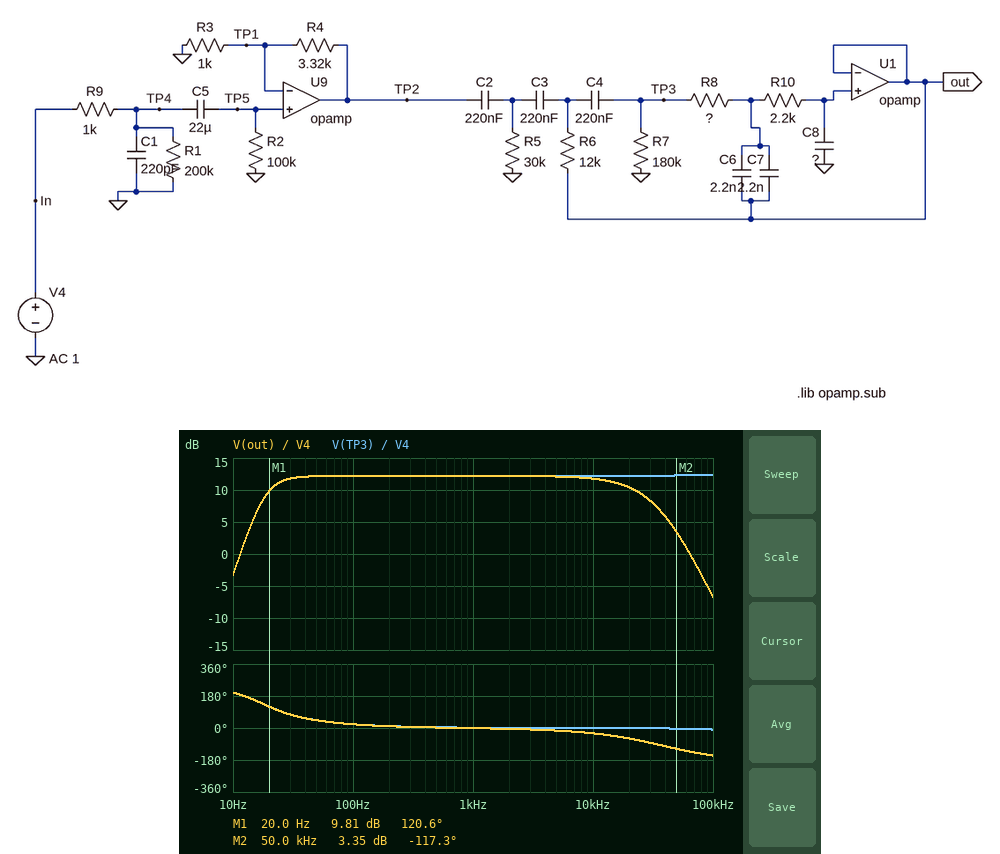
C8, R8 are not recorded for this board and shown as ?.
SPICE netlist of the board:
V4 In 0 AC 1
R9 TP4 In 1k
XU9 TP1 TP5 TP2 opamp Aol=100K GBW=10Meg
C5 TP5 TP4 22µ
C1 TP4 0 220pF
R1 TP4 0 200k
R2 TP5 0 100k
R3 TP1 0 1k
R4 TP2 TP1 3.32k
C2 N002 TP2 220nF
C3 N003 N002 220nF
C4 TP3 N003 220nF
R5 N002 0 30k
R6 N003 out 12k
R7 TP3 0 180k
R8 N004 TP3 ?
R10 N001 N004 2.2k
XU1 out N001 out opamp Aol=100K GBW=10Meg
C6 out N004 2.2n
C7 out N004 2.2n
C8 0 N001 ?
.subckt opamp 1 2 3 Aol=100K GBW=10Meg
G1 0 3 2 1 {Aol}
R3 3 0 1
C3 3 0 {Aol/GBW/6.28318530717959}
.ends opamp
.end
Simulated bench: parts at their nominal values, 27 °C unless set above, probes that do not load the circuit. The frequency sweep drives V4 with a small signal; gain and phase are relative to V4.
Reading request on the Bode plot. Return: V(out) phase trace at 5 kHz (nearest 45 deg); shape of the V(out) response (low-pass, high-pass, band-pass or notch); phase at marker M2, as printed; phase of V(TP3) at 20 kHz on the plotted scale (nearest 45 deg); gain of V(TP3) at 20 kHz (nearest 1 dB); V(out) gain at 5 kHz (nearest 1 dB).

0 deg
band-pass
-117.3 deg
0 deg
12 dB
12 dB
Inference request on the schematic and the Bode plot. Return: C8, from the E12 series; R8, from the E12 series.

2.7 nF
820 Ω
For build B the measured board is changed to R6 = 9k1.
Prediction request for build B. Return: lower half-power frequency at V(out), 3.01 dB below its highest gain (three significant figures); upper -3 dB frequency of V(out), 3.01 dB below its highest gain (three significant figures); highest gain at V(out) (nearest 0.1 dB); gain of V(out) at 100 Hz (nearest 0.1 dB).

20.6 Hz
23.9 kHz
12.7 dB
12.3 dB
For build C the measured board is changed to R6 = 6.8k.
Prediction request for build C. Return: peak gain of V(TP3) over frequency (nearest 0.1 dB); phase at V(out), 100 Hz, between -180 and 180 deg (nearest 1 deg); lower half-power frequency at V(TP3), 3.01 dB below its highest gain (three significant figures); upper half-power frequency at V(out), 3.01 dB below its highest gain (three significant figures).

13.5 dB
22 deg
23.4 Hz
19.6 kHz
